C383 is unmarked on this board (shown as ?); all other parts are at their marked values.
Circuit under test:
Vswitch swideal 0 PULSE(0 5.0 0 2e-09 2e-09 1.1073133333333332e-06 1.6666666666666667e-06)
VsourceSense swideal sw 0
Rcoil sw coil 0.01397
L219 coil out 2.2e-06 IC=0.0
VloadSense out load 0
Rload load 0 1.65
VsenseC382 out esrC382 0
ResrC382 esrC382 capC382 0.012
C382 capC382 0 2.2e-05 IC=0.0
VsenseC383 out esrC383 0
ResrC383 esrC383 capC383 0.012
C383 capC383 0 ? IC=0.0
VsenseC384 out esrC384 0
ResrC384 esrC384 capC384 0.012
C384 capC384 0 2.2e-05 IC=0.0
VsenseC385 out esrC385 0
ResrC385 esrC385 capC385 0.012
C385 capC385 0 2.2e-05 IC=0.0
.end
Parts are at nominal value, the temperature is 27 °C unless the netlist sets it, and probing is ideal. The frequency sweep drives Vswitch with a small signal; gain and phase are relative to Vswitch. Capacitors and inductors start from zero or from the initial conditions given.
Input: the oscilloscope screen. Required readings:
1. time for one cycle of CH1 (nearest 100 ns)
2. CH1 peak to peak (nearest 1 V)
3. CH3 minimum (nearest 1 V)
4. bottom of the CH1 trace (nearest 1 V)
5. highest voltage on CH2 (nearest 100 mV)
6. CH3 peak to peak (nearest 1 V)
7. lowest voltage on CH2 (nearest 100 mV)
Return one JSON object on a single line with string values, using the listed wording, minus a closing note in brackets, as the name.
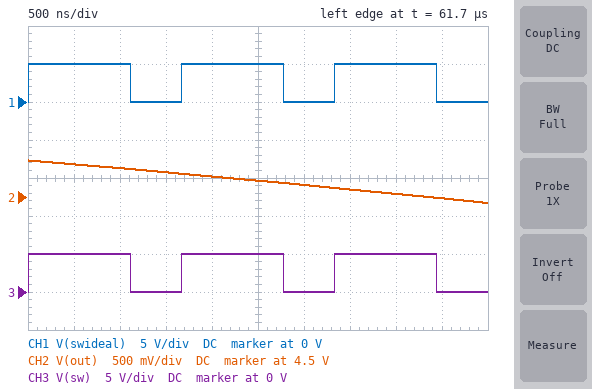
{"time for one cycle of CH1": "1.7 µs", "CH1 peak to peak": "5 V", "CH3 minimum": "0 V", "bottom of the CH1 trace": "0 V", "highest voltage on CH2": "5.0 V", "CH3 peak to peak": "5 V", "lowest voltage on CH2": "4.4 V"}
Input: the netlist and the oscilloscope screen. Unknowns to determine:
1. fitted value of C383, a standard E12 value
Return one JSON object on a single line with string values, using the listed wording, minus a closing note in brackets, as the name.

{"fitted value of C383, a standard E12 value": "47 µF"}
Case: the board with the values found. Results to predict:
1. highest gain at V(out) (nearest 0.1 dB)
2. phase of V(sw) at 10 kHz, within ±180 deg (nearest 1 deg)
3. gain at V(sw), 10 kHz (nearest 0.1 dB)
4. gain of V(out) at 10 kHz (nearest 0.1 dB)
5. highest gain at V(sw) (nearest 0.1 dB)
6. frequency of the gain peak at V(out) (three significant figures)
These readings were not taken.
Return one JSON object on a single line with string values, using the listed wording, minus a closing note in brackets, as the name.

{"highest gain at V(out)": "13.6 dB", "phase of V(sw) at 10 kHz, within ±180 deg": "0 deg", "gain at V(sw), 10 kHz": "0 dB", "gain of V(out) at 10 kHz": "13.6 dB", "highest gain at V(sw)": "0 dB", "frequency of the gain peak at V(out)": "10.0 kHz"}
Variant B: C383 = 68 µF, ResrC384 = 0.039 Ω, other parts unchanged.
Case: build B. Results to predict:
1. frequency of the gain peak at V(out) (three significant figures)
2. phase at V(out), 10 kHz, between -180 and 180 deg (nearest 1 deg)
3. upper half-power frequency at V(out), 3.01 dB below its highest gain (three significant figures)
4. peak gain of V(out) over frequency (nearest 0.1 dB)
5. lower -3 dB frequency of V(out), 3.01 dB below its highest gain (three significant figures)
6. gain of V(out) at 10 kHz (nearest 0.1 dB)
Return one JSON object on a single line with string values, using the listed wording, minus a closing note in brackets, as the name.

{"frequency of the gain peak at V(out)": "9.18 kHz", "phase at V(out), 10 kHz, between -180 and 180 deg": "-121 deg", "upper half-power frequency at V(out), 3.01 dB below its highest gain": "10.2 kHz", "peak gain of V(out) over frequency": "13.0 dB", "lower -3 dB frequency of V(out), 3.01 dB below its highest gain": "8.07 kHz", "gain of V(out) at 10 kHz": "10.8 dB"}
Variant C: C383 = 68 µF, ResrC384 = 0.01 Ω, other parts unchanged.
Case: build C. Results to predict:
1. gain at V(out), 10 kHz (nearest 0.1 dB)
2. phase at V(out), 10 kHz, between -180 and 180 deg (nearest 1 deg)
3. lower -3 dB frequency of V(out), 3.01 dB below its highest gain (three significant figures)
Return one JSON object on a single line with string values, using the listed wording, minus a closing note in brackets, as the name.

{"gain at V(out), 10 kHz": "11.0 dB", "phase at V(out), 10 kHz, between -180 and 180 deg": "-122 deg", "lower -3 dB frequency of V(out), 3.01 dB below its highest gain": "8.11 kHz"}
